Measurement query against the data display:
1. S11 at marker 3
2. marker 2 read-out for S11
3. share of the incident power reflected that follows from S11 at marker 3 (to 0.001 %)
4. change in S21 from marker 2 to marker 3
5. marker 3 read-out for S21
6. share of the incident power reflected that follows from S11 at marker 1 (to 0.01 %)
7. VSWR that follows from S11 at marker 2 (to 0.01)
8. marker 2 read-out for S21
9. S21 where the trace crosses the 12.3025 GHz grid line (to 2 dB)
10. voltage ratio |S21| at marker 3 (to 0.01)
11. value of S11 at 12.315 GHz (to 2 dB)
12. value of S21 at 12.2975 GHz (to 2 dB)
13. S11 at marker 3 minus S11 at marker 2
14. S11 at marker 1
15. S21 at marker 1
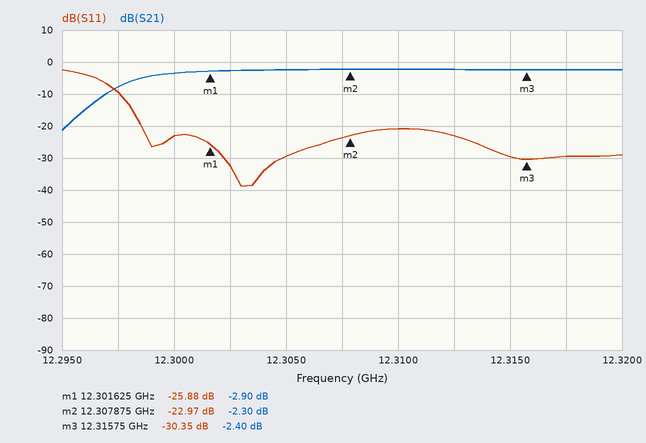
-30.35 dB
-22.97 dB
0.092 %
-0.10 dB
-2.40 dB
0.26 %
1.15
-2.30 dB
-2 dB
0.76
-30 dB
-8 dB
-7.38 dB
-25.88 dB
-2.90 dB
